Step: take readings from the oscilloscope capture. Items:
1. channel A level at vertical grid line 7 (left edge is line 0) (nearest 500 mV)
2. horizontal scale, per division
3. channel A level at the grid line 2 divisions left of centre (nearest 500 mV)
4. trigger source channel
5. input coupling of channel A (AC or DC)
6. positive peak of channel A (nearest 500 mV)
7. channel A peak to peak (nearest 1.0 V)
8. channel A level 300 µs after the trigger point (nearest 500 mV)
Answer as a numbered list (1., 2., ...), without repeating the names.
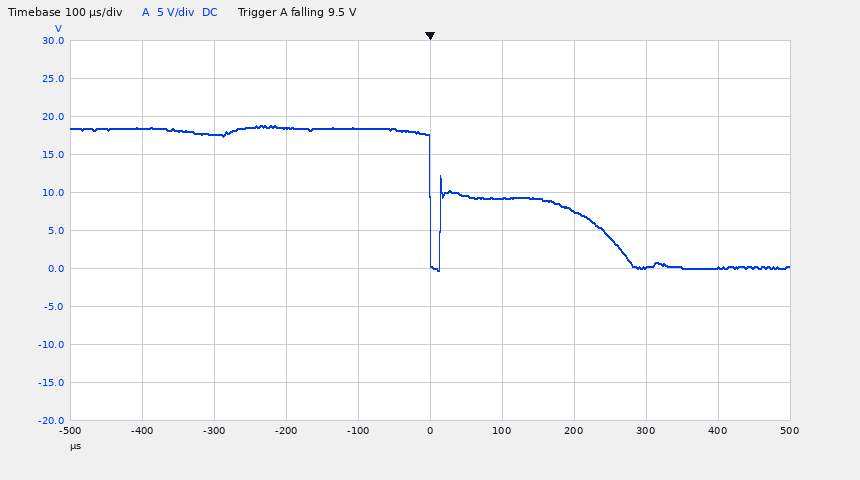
1. 7.5 V
2. 100 µs
3. 18.5 V
4. channel A
5. DC
6. 19.0 V
7. 19.0 V
8. 0.0 V
